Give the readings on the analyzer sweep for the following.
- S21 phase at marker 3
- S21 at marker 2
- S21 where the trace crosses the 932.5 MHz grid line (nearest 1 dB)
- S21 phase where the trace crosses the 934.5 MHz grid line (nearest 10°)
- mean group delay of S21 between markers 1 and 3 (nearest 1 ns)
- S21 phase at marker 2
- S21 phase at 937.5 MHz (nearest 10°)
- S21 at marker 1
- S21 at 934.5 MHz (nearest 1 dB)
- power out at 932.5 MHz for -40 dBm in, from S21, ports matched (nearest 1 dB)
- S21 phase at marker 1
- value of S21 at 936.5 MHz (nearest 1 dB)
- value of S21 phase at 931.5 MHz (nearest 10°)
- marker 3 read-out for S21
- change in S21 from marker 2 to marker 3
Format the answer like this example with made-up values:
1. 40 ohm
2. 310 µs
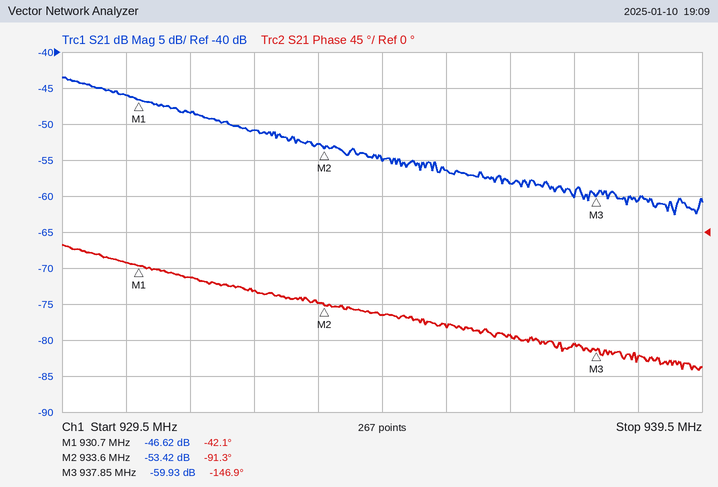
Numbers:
1. -146.9°
2. -53.42 dB
3. -51 dB
4. -100°
5. 41 ns
6. -91.3°
7. -140°
8. -46.62 dB
9. -55 dB
10. -91 dBm
11. -42.1°
12. -58 dB
13. -60°
14. -59.93 dB
15. -6.51 dB
